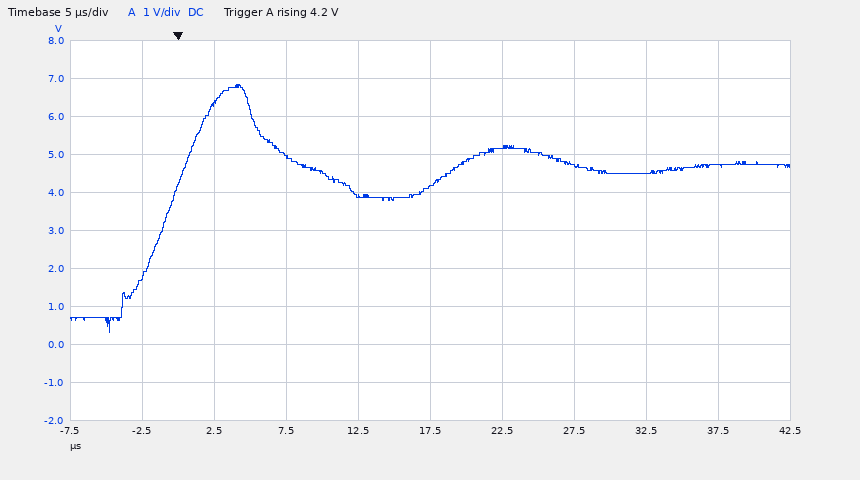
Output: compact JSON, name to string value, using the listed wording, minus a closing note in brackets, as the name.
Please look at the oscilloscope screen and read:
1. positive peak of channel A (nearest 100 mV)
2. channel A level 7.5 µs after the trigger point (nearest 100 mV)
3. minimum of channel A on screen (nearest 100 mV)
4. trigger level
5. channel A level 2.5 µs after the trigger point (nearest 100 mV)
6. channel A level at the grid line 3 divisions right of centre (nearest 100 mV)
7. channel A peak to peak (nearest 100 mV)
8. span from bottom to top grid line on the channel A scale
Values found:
{"positive peak of channel A": "6.8 V", "channel A level 7.5 µs after the trigger point": "5.0 V", "minimum of channel A on screen": "300 mV", "trigger level": "4.2 V", "channel A level 2.5 µs after the trigger point": "6.4 V", "channel A level at the grid line 3 divisions right of centre": "4.5 V", "channel A peak to peak": "6.5 V", "span from bottom to top grid line on the channel A scale": "10 V"}
